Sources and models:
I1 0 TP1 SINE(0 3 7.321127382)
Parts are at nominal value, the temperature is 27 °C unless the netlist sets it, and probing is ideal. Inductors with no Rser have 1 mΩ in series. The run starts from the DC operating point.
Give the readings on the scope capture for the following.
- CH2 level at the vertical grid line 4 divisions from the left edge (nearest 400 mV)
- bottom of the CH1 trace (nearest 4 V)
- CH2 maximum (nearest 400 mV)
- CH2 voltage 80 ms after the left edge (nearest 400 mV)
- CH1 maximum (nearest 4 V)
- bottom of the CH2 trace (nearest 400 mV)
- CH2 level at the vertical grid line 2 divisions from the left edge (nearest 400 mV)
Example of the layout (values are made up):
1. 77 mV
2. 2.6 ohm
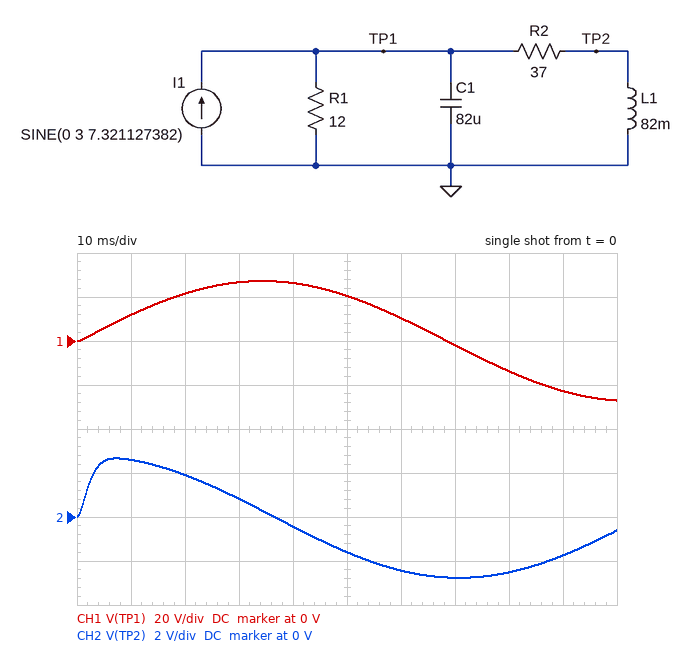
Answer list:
1. -400 mV
2. -28 V
3. 2.8 V
4. -2.4 V
5. 28 V
6. -2.8 V
7. 2.0 V
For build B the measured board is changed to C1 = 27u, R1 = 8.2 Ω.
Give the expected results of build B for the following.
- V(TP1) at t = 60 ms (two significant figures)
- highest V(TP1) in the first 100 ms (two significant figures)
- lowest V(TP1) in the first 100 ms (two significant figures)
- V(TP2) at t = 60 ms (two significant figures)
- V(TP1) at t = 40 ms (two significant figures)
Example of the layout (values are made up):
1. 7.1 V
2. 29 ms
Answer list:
1. 7.3 V
2. 20 V
3. -20 V
4. -1.8 V
5. 19 V
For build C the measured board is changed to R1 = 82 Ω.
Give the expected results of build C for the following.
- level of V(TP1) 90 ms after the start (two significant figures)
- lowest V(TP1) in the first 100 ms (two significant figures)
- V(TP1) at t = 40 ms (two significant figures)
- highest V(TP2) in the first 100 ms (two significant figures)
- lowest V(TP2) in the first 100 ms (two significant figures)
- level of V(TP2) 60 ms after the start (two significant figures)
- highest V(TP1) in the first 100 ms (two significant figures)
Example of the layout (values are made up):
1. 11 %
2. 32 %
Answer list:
1. -64 V
2. -76 V
3. 75 V
4. 8.1 V
5. -7.8 V
6. -6.8 V
7. 77 V
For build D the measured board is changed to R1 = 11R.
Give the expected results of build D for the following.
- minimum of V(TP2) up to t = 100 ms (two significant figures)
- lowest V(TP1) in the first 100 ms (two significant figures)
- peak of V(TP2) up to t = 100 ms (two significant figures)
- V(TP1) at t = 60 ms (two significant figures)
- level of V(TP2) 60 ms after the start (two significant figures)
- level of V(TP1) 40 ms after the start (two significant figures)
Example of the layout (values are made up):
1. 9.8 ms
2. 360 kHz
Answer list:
1. -2.6 V
2. -25 V
3. 2.5 V
4. 9.7 V
5. -2.3 V
6. 25 V
